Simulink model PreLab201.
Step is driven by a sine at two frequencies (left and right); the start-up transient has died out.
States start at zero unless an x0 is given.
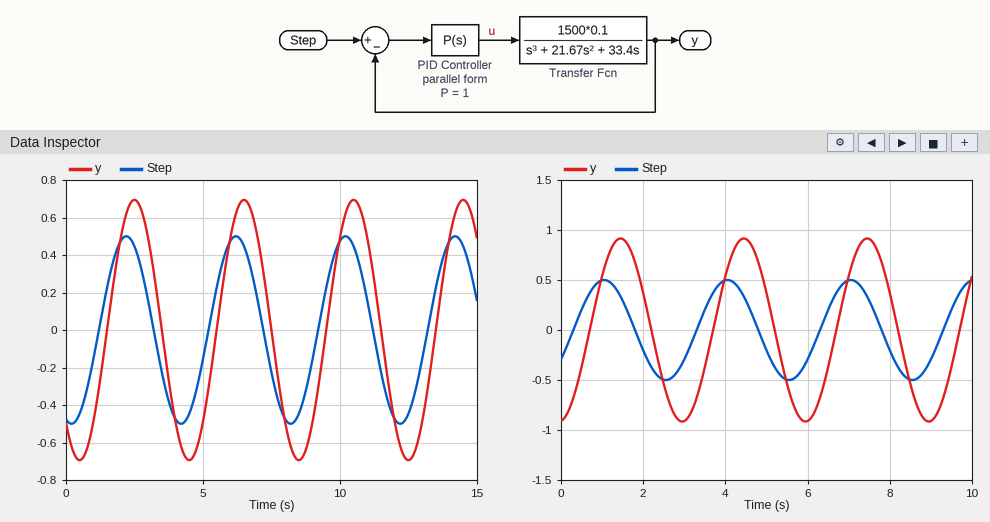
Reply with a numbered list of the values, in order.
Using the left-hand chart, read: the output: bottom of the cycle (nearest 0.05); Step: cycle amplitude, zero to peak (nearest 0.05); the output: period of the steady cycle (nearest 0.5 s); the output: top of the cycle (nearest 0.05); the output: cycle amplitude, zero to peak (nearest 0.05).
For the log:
1. -0.70
2. 0.50
3. 4.0 s
4. 0.70
5. 0.70
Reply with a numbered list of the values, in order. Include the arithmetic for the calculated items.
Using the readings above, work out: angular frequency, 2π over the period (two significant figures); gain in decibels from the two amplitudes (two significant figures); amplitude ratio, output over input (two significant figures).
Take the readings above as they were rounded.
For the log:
1. 2π / 4 = 1.6 rad/s
2. 20 log10(0.7 / 0.5) = 2.9 dB
3. 0.7 / 0.5 = 1.4
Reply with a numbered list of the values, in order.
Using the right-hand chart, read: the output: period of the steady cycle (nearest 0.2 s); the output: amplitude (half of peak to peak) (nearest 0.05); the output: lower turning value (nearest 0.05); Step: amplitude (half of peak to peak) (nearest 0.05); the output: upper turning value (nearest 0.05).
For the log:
1. 3.0 s
2. 0.90
3. -0.90
4. 0.50
5. 0.90
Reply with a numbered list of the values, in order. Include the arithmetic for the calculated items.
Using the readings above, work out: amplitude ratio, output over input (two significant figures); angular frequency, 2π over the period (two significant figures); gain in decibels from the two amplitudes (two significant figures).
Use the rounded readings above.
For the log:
1. 0.9 / 0.5 = 1.8
2. 2π / 3 = 2.1 rad/s
3. 20 log10(0.9 / 0.5) = 5.1 dB
